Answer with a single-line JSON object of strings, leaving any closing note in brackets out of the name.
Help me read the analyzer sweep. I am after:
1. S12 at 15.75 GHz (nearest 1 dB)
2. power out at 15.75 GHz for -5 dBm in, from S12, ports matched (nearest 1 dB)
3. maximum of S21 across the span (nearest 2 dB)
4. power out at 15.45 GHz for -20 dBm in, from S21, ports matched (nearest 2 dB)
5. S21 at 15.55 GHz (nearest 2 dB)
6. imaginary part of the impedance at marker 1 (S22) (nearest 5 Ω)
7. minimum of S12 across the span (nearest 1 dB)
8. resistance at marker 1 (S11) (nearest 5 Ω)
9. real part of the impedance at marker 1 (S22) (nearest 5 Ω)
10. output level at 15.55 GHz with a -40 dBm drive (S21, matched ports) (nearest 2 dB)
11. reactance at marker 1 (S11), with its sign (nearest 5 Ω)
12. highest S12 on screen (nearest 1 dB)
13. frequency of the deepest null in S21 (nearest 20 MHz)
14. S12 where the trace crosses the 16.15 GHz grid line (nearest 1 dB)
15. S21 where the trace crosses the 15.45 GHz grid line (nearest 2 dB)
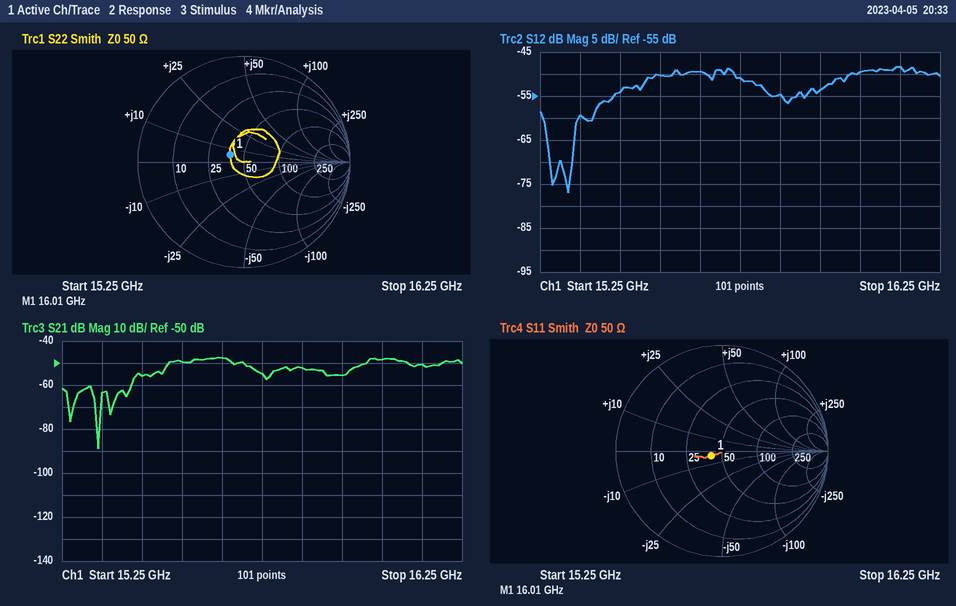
{"S12 at 15.75 GHz": "-51 dB", "power out at 15.75 GHz for -5 dBm in, from S12, ports matched": "-56 dBm", "maximum of S21 across the span": "-48 dB", "power out at 15.45 GHz for -20 dBm in, from S21, ports matched": "-76 dBm", "S21 at 15.55 GHz": "-50 dB", "imaginary part of the impedance at marker 1 (S22)": "+5 Ω", "minimum of S12 across the span": "-77 dB", "resistance at marker 1 (S11)": "40 Ω", "real part of the impedance at marker 1 (S22)": "40 Ω", "output level at 15.55 GHz with a -40 dBm drive (S21, matched ports)": "-90 dBm", "reactance at marker 1 (S11), with its sign": "-5 Ω", "highest S12 on screen": "-48 dB", "frequency of the deepest null in S21": "15.34 GHz", "S12 where the trace crosses the 16.15 GHz grid line": "-48 dB", "S21 where the trace crosses the 15.45 GHz grid line": "-56 dB"}
